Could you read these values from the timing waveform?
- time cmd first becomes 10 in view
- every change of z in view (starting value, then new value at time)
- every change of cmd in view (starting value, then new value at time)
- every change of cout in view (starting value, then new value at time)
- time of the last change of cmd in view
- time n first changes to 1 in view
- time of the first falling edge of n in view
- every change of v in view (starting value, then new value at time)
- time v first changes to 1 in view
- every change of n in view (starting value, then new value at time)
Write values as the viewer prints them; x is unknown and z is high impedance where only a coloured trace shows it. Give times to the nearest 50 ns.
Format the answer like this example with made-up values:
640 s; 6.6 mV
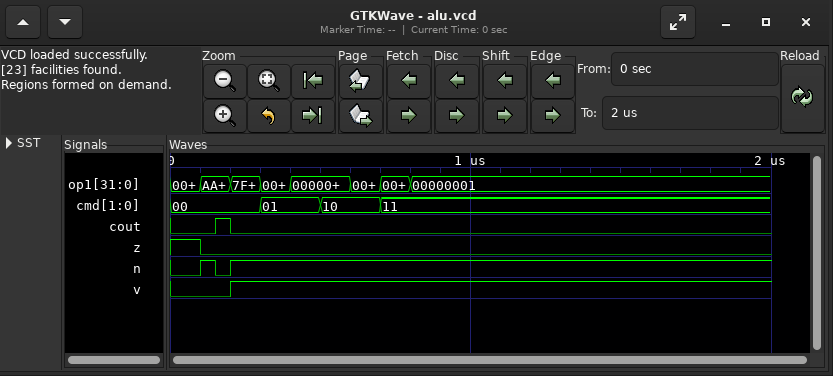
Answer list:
500 ns; 1, 0 at 100 ns; 00, 01 at 300 ns, 10 at 500 ns, 11 at 700 ns; 0, 1 at 150 ns, 0 at 200 ns; 700 ns; 100 ns; 150 ns; 0, 1 at 200 ns; 200 ns; 0, 1 at 100 ns, 0 at 150 ns, 1 at 200 ns
